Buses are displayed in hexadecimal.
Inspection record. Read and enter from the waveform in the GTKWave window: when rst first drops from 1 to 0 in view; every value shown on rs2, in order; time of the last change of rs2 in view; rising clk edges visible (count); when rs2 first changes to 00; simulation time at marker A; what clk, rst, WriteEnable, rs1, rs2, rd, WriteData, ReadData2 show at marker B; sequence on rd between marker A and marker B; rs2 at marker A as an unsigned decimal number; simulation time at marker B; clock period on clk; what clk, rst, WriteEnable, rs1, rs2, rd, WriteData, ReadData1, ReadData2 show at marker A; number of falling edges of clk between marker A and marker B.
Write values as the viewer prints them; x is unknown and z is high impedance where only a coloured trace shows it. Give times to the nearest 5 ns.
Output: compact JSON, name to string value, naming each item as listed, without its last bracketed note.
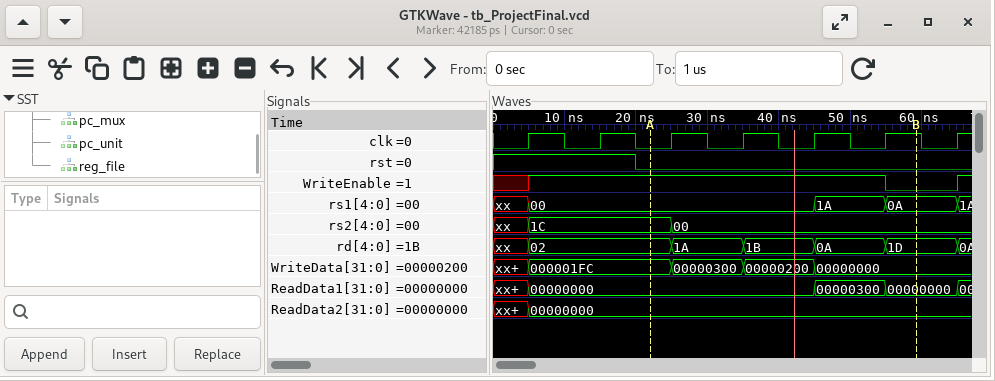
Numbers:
{"when rst first drops from 1 to 0 in view": "20 ns", "every value shown on rs2, in order": "xx, 1C, 00", "time of the last change of rs2 in view": "25 ns", "rising clk edges visible": "7", "when rs2 first changes to 00": "25 ns", "simulation time at marker A": "20 ns", "what clk, rst, WriteEnable, rs1, rs2, rd, WriteData, ReadData2 show at marker B": "clk=1, rst=0, WriteEnable=0, rs1=0A, rs2=00, rd=1D, WriteData=00000000, ReadData2=00000000", "sequence on rd between marker A and marker B": "02, 1A, 1B, 0A, 1D", "rs2 at marker A as an unsigned decimal number": "28", "simulation time at marker B": "60 ns", "clock period on clk": "10 ns", "what clk, rst, WriteEnable, rs1, rs2, rd, WriteData, ReadData1, ReadData2 show at marker A": "clk=0, rst=0, WriteEnable=1, rs1=00, rs2=1C, rd=02, WriteData=000001FC, ReadData1=00000000, ReadData2=00000000", "number of falling edges of clk between marker A and marker B": "3"}
